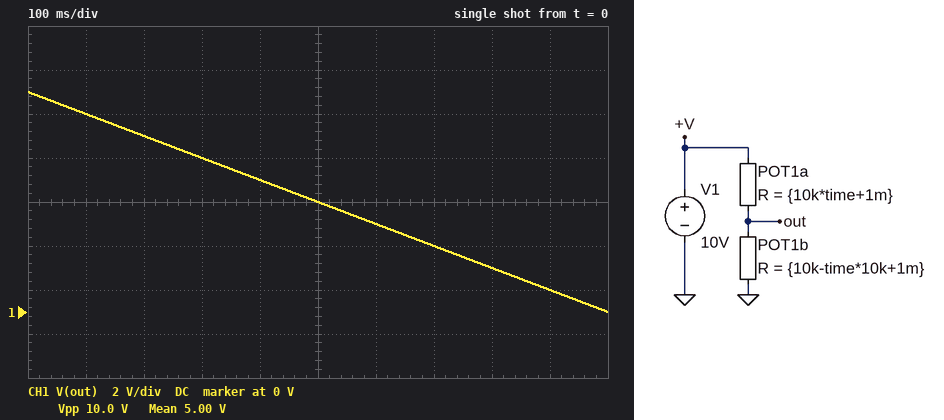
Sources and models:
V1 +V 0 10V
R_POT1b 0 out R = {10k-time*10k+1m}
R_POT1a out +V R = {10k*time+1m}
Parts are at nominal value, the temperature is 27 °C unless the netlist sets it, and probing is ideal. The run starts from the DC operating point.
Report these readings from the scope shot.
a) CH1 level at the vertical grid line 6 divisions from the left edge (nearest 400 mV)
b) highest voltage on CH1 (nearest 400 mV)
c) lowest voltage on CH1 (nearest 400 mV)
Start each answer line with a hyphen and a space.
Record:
- 4.0 V
- 10.0 V
- 0 V
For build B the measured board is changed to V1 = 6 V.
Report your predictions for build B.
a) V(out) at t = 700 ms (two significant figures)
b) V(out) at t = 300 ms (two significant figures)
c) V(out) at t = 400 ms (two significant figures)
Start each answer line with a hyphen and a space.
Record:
- 1.8 V
- 4.2 V
- 3.6 V
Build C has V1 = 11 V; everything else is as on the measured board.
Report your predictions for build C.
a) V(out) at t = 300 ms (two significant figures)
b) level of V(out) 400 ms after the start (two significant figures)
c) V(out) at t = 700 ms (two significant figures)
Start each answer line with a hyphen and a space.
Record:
- 7.7 V
- 6.6 V
- 3.3 V
